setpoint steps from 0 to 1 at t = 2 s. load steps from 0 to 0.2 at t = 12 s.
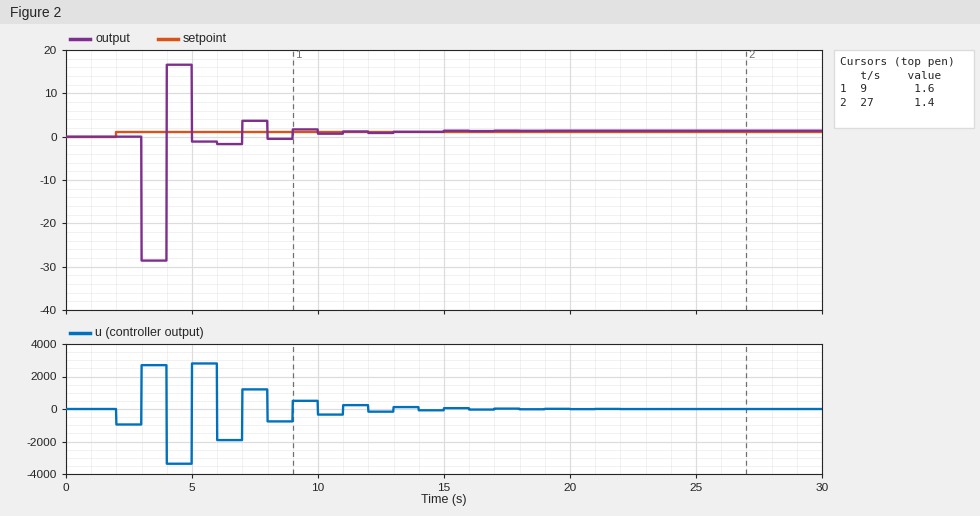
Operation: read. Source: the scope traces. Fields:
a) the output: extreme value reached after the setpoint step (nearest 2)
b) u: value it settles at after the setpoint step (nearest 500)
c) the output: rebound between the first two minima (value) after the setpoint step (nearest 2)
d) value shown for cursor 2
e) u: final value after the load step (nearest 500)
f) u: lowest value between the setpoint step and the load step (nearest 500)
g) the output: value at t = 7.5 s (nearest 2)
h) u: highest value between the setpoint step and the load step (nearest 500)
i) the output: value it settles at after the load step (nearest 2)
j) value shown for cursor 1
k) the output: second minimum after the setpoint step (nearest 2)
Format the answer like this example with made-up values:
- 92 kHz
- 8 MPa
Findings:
- -28
- 0
- 16
- 1.4
- 0
- -3500
- 4
- 3000
- 2
- 1.6
- -2
